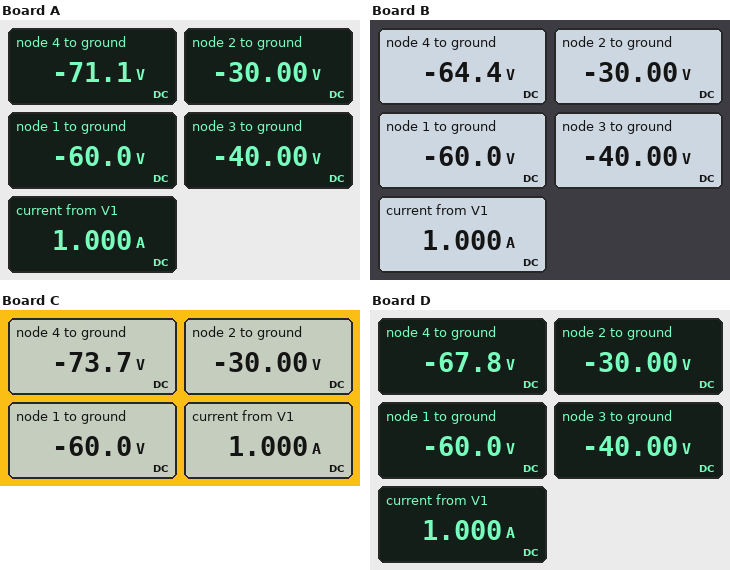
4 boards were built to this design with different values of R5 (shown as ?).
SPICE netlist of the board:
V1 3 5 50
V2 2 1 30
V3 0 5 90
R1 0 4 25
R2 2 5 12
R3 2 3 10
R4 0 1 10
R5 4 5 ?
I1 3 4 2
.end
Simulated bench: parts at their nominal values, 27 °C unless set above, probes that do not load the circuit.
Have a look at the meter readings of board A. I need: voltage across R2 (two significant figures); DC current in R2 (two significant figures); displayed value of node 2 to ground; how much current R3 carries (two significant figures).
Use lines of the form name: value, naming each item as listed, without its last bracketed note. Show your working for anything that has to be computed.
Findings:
voltage across R2: -30 V - (-90 V) = 60 V
DC current in R2: (-30 V - (-90 V)) / 12 Ω = 5.0 A
displayed value of node 2 to ground: -30.00 V
how much current R3 carries: (-30 V - (-40 V)) / 10 Ω = 1.0 A
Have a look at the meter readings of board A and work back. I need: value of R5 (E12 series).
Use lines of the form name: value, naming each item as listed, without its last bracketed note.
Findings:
value of R5: 3.9 Ω
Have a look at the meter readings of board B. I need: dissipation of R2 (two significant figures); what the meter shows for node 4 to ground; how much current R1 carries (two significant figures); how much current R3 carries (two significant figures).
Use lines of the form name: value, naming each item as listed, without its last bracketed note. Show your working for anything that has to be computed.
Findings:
dissipation of R2: (-30 V - (-90 V))^2 / 12 Ω = 300 W
what the meter shows for node 4 to ground: -64.4 V
how much current R1 carries: (0 V - (-64.4 V)) / 25 Ω = 2.6 A
how much current R3 carries: (-30 V - (-40 V)) / 10 Ω = 1.0 A
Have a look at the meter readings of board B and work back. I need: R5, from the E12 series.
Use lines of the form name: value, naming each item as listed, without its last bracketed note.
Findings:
R5, from the E12 series: 5.6 Ω
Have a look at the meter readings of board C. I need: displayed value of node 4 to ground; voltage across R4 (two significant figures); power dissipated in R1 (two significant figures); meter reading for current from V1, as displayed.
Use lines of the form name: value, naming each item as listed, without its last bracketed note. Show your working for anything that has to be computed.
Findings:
displayed value of node 4 to ground: -73.7 V
voltage across R4: 0 V - (-60 V) = 60 V
power dissipated in R1: (0 V - (-73.7 V))^2 / 25 Ω = 220 W
meter reading for current from V1, as displayed: 1.000 A
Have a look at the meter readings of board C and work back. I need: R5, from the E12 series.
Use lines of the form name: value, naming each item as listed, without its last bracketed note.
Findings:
R5, from the E12 series: 3.3 Ω
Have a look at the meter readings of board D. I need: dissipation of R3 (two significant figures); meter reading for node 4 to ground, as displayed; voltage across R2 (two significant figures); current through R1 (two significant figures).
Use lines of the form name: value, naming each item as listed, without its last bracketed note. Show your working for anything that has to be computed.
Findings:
dissipation of R3: (-30 V - (-40 V))^2 / 10 Ω = 10 W
meter reading for node 4 to ground, as displayed: -67.8 V
voltage across R2: -30 V - (-90 V) = 60 V
current through R1: (0 V - (-67.8 V)) / 25 Ω = 2.7 A
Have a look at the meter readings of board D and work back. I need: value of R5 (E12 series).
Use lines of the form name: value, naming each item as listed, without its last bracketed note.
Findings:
value of R5: 4.7 Ω
